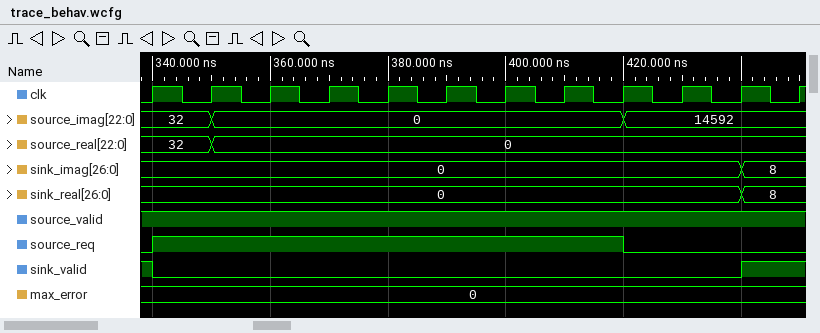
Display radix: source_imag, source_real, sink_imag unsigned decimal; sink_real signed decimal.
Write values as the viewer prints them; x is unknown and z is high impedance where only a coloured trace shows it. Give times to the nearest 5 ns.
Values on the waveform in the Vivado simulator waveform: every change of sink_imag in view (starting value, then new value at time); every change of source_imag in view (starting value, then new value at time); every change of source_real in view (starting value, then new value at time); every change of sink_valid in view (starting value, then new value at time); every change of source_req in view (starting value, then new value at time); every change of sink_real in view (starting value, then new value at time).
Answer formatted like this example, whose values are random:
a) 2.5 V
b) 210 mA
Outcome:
a) 0, 8 at 440 ns
b) 32, 0 at 350 ns, 14592 at 420 ns
c) 32, 0 at 350 ns
d) 1, 0 at 340 ns, 1 at 440 ns
e) 0, 1 at 340 ns, 0 at 420 ns
f) 0, 8 at 440 ns
